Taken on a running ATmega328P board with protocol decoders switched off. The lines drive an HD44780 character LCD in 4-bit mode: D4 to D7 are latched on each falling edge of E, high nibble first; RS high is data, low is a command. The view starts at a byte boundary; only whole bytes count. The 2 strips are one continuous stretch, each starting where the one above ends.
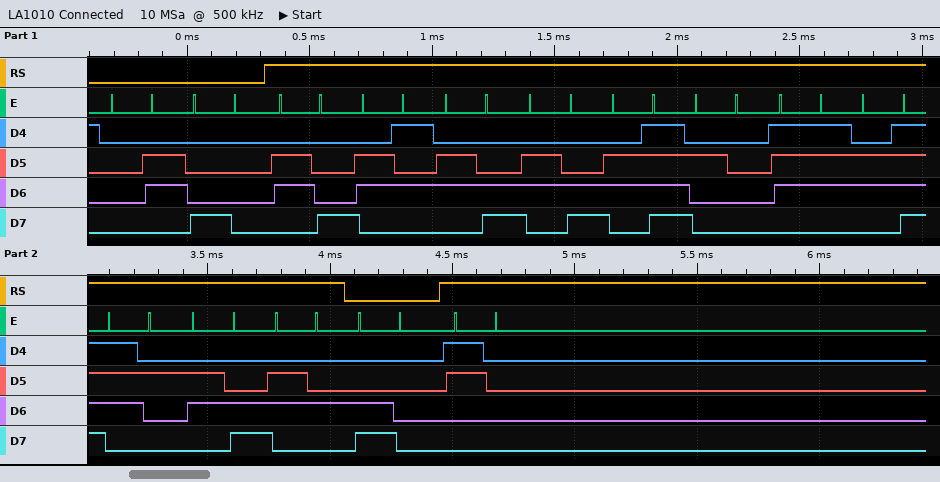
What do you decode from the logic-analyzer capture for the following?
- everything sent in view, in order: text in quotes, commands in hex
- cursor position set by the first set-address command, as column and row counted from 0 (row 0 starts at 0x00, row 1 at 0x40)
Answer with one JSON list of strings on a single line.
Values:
["0x06 0x80 \"hello world\" 0xC0 \"0\"", "column 0, row 0"]
